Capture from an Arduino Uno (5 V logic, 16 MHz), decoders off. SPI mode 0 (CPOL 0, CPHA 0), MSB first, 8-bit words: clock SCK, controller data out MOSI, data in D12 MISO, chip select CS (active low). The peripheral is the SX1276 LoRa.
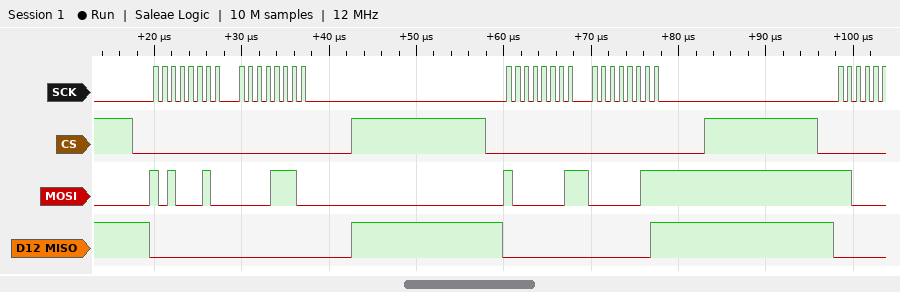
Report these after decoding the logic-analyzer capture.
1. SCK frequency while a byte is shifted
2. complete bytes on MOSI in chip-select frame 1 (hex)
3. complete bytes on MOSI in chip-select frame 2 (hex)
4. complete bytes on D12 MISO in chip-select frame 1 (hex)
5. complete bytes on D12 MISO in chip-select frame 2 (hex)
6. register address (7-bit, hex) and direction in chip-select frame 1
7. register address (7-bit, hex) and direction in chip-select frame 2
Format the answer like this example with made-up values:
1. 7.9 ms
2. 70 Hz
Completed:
1. 1 MHz
2. 0xA2 0x0E
3. 0x81 0x03
4. 0x00 0x00
5. 0x00 0x01
6. 0x22 write
7. 0x01 write
